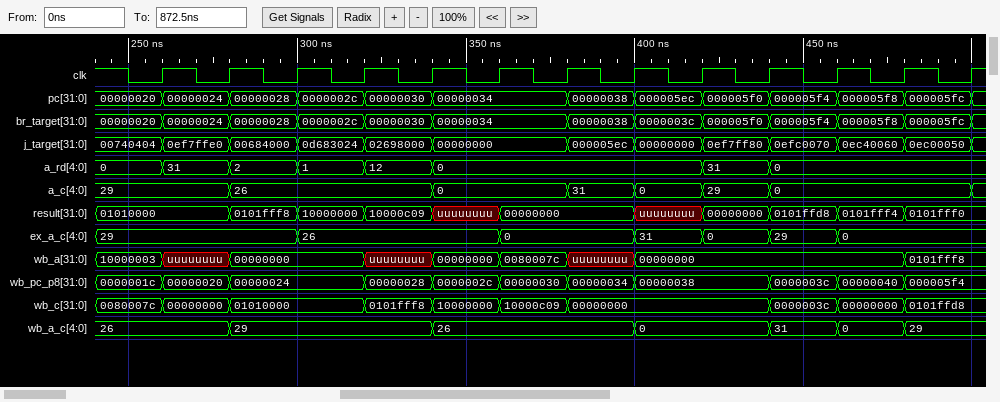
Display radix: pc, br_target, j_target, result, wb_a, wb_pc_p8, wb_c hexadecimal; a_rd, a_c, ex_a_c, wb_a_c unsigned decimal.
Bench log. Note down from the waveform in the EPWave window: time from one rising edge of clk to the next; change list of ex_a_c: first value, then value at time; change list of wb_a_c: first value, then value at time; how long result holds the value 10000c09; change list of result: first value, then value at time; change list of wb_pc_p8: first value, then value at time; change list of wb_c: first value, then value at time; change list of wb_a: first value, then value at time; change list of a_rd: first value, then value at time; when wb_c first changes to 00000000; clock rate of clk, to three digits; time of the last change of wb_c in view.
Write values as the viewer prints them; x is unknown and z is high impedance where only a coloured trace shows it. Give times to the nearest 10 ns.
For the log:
20 ns
29, 26 at 300 ns, 0 at 360 ns, 31 at 400 ns, 0 at 420 ns, 29 at 440 ns, 0 at 460 ns
26, 29 at 280 ns, 26 at 340 ns, 0 at 400 ns, 31 at 440 ns, 0 at 460 ns, 29 at 480 ns
20 ns
01010000, 0101fff8 at 280 ns, 10000000 at 300 ns, 10000c09 at 320 ns, uuuuuuuu at 340 ns, 00000000 at 360 ns, uuuuuuuu at 400 ns, 00000000 at 420 ns, 0101ffd8 at 440 ns, 0101fff4 at 460 ns, 0101fff0 at 480 ns
0000001c, 00000020 at 260 ns, 00000024 at 280 ns, 00000028 at 320 ns, 0000002c at 340 ns, 00000030 at 360 ns, 00000034 at 380 ns, 00000038 at 400 ns, 0000003c at 440 ns, 00000040 at 460 ns, 000005f4 at 480 ns
0080007c, 00000000 at 260 ns, 01010000 at 280 ns, 0101fff8 at 320 ns, 10000000 at 340 ns, 10000c09 at 360 ns, 00000000 at 380 ns, 0000003c at 440 ns, 00000000 at 460 ns, 0101ffd8 at 480 ns
10000003, uuuuuuuu at 260 ns, 00000000 at 280 ns, uuuuuuuu at 320 ns, 00000000 at 340 ns, 0080007c at 360 ns, uuuuuuuu at 380 ns, 00000000 at 400 ns, 0101fff8 at 480 ns
0, 31 at 260 ns, 2 at 280 ns, 1 at 300 ns, 12 at 320 ns, 0 at 340 ns, 31 at 420 ns, 0 at 440 ns
260 ns
50.0 MHz
480 ns
